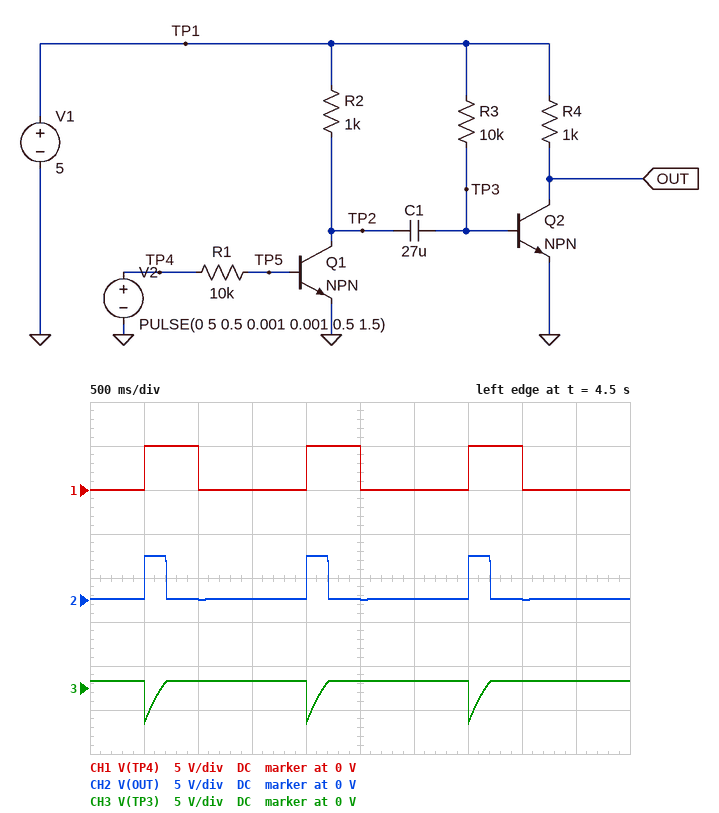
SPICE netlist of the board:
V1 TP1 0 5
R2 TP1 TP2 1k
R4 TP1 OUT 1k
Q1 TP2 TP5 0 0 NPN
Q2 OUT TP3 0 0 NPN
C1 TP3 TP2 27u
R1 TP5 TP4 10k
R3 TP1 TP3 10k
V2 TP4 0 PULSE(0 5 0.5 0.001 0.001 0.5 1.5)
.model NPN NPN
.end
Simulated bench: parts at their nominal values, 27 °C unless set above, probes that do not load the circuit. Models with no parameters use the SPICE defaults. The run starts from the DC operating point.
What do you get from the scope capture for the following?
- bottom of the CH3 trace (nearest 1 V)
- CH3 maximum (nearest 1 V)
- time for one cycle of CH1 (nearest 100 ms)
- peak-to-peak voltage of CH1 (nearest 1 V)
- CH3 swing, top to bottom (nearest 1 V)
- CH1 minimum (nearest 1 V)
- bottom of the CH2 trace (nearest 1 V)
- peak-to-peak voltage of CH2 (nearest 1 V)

-4 V
1 V
1.5 s
5 V
5 V
0 V
0 V
5 V
